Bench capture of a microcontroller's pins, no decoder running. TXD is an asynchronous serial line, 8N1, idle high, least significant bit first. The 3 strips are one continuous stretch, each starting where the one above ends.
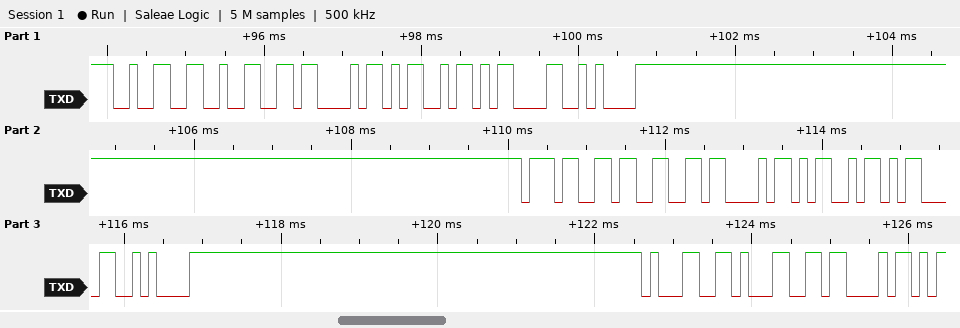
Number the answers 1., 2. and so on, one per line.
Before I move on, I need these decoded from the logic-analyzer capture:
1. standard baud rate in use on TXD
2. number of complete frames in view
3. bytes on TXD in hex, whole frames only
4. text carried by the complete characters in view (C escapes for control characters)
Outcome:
1. 9600 baud
2. 15
3. 32 32 43 4D 0D 0A 37 33 43 4D 0D 0A 31 31 43
4. "22CM\r\n73CM\r\n11C"
